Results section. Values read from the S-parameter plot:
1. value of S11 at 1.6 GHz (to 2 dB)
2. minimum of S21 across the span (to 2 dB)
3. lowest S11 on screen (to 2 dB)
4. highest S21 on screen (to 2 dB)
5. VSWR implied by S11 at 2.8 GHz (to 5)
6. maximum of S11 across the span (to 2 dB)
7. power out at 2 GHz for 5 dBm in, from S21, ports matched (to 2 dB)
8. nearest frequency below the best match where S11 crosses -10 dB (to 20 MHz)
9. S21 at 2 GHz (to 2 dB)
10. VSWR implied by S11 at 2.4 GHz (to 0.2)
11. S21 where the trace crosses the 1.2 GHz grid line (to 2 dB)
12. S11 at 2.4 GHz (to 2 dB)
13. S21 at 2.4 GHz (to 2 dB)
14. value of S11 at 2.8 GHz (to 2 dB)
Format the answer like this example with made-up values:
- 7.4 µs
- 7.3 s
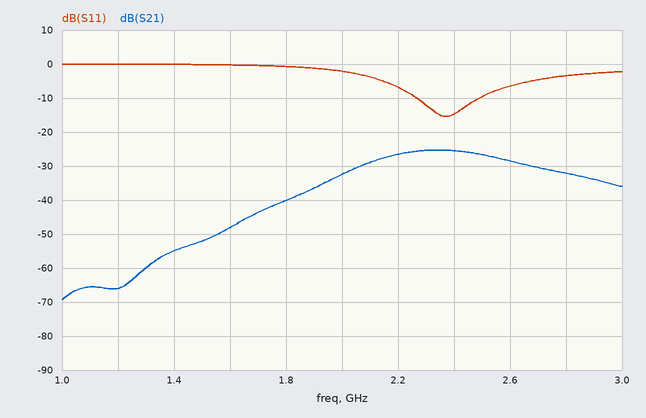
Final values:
- 0 dB
- -70 dB
- -16 dB
- -26 dB
- 5
- 0 dB
- -28 dBm
- 2.26 GHz
- -32 dB
- 1.4
- -66 dB
- -14 dB
- -26 dB
- -4 dB
